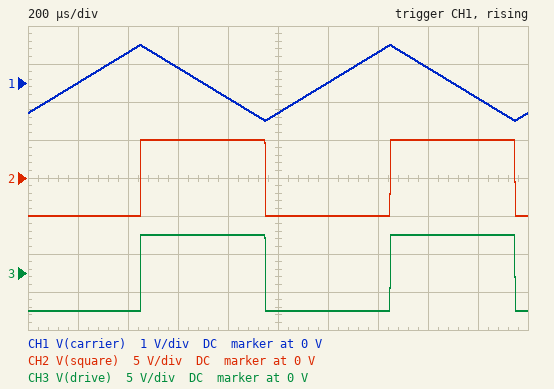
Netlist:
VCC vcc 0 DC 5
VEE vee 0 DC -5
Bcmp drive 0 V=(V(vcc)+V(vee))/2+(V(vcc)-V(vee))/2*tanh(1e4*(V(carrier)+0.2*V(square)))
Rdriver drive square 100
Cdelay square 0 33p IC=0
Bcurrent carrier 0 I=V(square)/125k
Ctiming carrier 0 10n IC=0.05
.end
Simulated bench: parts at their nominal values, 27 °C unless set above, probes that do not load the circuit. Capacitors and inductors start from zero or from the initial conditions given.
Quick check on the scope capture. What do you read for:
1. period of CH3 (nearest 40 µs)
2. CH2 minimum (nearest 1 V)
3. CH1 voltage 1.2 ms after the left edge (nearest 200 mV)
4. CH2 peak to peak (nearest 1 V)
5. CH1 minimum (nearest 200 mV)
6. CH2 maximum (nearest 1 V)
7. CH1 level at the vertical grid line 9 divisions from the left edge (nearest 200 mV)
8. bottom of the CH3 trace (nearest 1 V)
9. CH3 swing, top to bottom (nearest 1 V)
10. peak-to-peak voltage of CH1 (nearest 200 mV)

1.00 ms
-5 V
0 V
10 V
-1.0 V
5 V
-400 mV
-5 V
10 V
2.0 V
